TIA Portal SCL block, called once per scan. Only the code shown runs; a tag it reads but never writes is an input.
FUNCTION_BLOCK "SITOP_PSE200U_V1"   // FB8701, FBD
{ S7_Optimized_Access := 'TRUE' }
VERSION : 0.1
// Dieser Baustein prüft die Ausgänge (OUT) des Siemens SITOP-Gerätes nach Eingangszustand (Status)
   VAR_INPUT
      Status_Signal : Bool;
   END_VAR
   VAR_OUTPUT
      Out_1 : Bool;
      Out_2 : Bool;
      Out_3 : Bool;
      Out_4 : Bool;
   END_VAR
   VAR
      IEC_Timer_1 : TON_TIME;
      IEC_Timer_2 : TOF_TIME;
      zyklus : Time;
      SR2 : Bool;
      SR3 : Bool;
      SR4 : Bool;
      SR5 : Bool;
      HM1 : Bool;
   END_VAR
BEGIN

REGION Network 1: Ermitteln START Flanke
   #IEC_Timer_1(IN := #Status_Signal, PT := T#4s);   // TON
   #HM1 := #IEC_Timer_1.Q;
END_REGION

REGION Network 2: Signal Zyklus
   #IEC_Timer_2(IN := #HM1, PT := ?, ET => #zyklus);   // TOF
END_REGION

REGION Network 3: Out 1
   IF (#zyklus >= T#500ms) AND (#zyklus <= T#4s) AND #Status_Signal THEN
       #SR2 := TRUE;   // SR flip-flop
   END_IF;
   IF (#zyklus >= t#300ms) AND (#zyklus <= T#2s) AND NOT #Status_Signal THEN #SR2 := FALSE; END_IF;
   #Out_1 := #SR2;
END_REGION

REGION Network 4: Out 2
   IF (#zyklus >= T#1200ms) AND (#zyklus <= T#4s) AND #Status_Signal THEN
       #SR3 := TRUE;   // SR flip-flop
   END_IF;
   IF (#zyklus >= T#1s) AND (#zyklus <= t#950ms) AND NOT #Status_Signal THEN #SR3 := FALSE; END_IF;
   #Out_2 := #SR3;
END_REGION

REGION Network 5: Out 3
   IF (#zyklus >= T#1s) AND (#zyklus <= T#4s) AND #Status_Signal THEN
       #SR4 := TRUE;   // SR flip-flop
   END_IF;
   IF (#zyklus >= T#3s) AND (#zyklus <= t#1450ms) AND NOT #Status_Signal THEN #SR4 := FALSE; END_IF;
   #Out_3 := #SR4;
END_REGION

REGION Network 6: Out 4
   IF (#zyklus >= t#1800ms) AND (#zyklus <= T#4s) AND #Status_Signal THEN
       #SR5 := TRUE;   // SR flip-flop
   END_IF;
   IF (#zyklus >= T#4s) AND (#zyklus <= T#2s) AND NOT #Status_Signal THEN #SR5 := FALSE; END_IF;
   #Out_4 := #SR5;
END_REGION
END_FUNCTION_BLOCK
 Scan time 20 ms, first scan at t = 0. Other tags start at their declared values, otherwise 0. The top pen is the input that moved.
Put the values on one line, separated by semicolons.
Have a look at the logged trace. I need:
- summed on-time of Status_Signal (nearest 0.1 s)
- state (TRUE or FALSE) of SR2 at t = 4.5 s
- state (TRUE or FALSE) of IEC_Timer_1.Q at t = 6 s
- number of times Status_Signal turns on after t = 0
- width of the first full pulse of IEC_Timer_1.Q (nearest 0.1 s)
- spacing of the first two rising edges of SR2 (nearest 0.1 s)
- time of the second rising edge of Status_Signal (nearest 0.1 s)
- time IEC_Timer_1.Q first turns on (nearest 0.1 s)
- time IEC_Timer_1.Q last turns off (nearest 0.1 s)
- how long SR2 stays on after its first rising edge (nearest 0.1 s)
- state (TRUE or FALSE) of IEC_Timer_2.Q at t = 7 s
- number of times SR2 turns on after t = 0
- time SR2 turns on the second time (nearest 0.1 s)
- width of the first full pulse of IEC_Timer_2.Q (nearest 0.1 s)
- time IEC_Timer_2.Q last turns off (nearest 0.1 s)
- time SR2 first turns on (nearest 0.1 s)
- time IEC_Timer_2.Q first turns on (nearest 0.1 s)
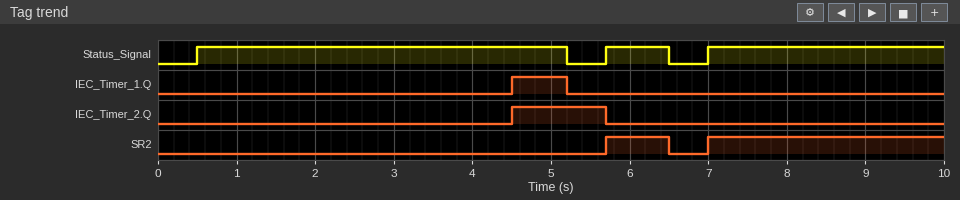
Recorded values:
8.5 s; FALSE; FALSE; 3; 0.7 s; 1.3 s; 5.7 s; 4.5 s; 5.2 s; 0.8 s; FALSE; 2; 7.0 s; 1.2 s; 5.7 s; 5.7 s; 4.5 s
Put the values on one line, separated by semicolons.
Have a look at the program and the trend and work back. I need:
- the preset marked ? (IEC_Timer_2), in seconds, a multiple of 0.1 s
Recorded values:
0.5 s
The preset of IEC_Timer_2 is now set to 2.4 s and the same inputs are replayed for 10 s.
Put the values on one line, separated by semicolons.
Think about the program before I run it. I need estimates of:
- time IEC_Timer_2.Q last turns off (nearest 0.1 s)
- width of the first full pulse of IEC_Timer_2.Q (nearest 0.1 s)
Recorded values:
7.6 s; 3.1 s
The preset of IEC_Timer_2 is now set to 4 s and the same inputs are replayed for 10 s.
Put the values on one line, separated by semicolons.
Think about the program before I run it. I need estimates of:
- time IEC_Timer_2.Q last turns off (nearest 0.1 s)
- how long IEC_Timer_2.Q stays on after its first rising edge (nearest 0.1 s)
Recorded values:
9.2 s; 4.7 s
